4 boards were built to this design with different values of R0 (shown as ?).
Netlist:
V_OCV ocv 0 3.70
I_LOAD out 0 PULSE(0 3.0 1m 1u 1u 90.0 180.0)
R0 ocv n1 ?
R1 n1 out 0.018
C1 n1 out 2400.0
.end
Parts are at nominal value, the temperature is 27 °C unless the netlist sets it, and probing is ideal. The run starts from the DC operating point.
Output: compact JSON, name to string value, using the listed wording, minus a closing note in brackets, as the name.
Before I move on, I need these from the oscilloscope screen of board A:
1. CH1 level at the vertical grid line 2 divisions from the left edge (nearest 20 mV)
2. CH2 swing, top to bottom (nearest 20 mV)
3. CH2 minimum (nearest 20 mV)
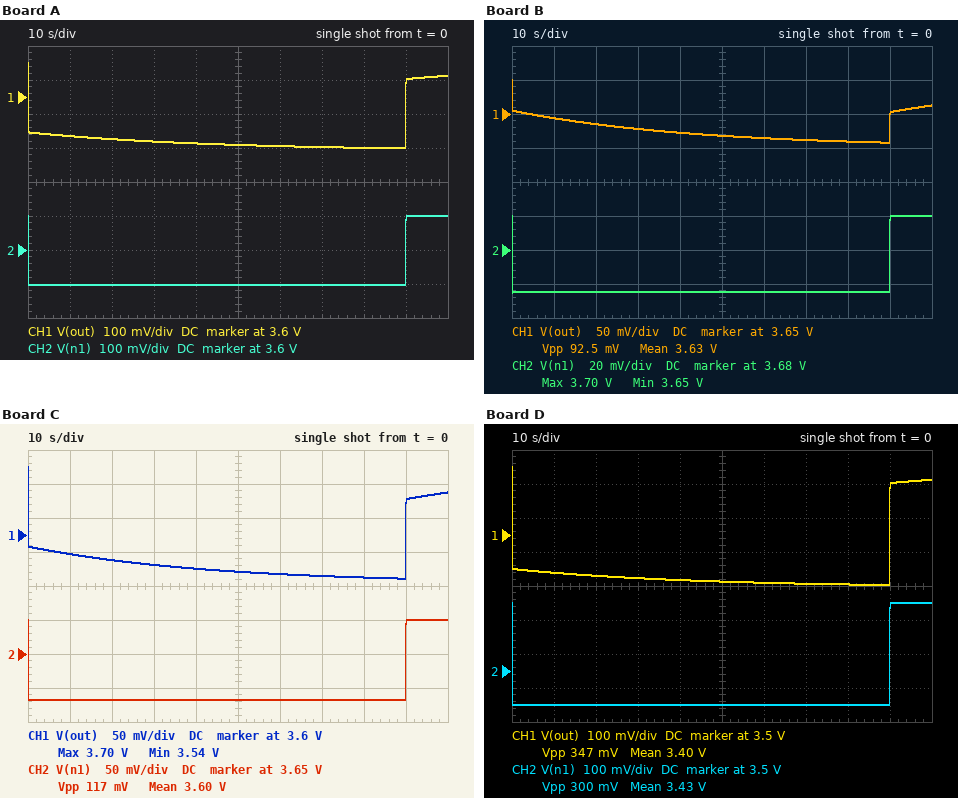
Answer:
{"CH1 level at the vertical grid line 2 divisions from the left edge": "3.48 V", "CH2 swing, top to bottom": "200 mV", "CH2 minimum": "3.50 V"}
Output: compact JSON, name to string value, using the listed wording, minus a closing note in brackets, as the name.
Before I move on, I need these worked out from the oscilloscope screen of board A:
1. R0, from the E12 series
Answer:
{"R0, from the E12 series": "0.068 Ω"}
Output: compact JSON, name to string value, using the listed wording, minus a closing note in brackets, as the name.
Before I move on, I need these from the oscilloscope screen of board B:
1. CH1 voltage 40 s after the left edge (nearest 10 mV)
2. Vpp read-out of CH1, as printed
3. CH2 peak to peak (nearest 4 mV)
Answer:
{"CH1 voltage 40 s after the left edge": "3.62 V", "Vpp read-out of CH1, as printed": "92.5 mV", "CH2 peak to peak": "44 mV"}
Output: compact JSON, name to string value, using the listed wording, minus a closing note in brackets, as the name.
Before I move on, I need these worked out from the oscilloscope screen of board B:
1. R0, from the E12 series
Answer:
{"R0, from the E12 series": "0.015 Ω"}
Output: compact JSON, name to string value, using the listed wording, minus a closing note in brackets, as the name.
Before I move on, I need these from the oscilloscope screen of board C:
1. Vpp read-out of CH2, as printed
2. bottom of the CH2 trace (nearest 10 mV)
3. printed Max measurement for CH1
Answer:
{"Vpp read-out of CH2, as printed": "117 mV", "bottom of the CH2 trace": "3.58 V", "printed Max measurement for CH1": "3.70 V"}
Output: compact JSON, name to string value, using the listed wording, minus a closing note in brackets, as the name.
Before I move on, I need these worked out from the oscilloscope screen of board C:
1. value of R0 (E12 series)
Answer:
{"value of R0": "0.039 Ω"}
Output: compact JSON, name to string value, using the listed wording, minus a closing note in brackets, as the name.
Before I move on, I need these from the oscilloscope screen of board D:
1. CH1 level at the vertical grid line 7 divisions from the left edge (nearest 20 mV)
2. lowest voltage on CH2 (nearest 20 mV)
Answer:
{"CH1 level at the vertical grid line 7 divisions from the left edge": "3.36 V", "lowest voltage on CH2": "3.40 V"}
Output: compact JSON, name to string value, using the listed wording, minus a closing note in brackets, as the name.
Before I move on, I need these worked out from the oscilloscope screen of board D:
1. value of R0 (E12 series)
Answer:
{"value of R0": "0.1 Ω"}
